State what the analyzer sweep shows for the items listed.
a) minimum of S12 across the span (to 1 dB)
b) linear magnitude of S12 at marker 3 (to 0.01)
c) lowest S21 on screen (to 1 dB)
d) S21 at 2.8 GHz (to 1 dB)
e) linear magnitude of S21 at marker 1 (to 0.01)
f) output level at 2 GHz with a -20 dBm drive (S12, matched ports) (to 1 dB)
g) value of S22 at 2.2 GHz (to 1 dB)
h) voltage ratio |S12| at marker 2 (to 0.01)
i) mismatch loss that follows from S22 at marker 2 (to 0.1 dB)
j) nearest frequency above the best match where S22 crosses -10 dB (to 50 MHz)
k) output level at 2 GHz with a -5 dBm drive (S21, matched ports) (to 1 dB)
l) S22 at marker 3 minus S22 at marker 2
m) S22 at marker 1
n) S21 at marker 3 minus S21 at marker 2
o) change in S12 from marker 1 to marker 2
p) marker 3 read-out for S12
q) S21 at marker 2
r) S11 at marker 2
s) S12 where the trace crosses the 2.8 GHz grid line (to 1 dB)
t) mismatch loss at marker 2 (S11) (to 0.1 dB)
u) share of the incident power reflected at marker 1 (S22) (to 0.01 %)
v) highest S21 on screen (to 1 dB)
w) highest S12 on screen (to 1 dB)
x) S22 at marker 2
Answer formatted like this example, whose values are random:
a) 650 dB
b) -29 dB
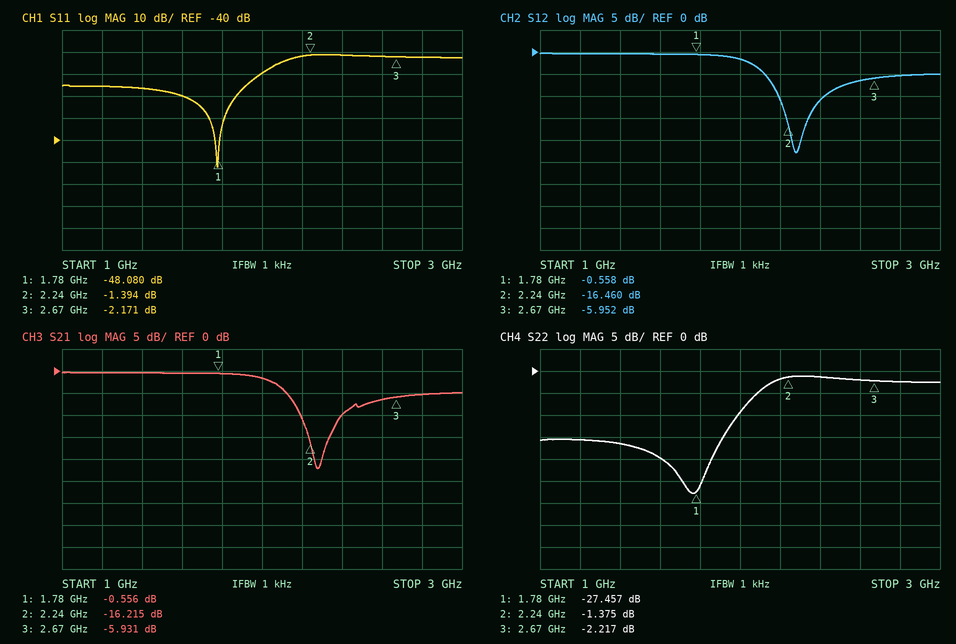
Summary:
a) -23 dB
b) 0.50
c) -22 dB
d) -5 dB
e) 0.94
f) -22 dBm
g) -2 dB
h) 0.15
i) 5.7 dB
j) 2.00 GHz
k) -7 dBm
l) -0.842 dB
m) -27.457 dB
n) 10.284 dB
o) -15.902 dB
p) -5.952 dB
q) -16.215 dB
r) -1.394 dB
s) -5 dB
t) 5.6 dB
u) 0.18 %
v) 0 dB
w) 0 dB
x) -1.375 dB
